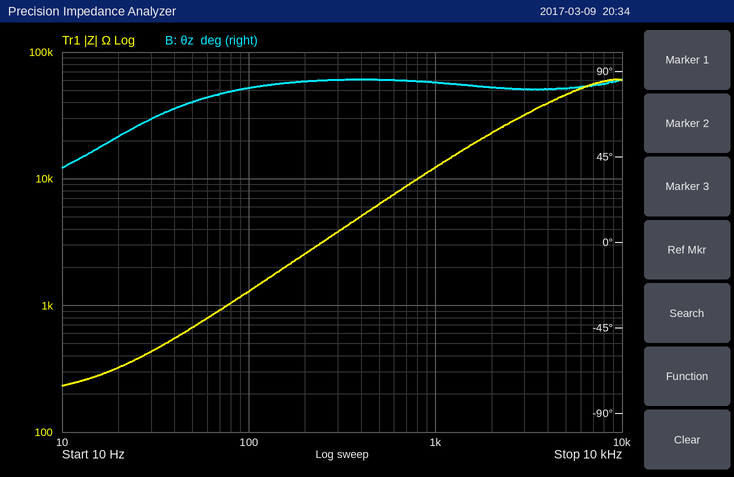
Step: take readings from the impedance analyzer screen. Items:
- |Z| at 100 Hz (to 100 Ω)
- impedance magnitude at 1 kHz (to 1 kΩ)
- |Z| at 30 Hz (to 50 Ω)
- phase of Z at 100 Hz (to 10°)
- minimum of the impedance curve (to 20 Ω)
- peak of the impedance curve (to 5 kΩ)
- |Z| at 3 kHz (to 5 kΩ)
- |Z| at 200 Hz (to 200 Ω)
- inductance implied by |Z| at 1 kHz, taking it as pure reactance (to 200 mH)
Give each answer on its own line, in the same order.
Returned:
1.3 kΩ
12 kΩ
450 Ω
80°
240 Ω
60 kΩ
30 kΩ
2.6 kΩ
2.0 H
